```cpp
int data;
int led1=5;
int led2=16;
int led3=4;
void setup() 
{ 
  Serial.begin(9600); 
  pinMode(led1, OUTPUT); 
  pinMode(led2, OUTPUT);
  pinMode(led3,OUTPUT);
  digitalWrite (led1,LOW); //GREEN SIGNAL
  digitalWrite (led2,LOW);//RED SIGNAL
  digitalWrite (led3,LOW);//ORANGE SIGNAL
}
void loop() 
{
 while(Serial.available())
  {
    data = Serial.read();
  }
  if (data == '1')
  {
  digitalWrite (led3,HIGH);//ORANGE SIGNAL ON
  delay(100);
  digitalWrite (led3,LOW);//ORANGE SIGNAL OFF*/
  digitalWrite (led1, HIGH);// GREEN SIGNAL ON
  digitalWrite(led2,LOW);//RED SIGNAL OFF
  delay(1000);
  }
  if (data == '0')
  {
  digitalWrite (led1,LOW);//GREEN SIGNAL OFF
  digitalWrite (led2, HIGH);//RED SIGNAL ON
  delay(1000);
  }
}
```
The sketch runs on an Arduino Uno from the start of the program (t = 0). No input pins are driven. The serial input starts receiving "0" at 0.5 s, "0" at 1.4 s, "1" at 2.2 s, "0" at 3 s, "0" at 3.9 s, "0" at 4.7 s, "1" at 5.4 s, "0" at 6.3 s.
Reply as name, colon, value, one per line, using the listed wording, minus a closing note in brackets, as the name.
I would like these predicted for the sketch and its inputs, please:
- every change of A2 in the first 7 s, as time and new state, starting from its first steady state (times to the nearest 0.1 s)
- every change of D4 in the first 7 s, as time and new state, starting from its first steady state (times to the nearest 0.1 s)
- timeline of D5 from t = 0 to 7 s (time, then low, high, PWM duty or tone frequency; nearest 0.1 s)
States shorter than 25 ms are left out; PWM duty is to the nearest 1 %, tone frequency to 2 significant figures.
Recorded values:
every change of A2 in the first 7 s, as time and new state, starting from its first steady state: 0 s low; 0.5 s high; 2.6 s low; 3.6 s high; 5.7 s low; 6.7 s high
every change of D4 in the first 7 s, as time and new state, starting from its first steady state: 0 s low; 2.5 s high; 2.6 s low; 5.6 s high; 5.7 s low
timeline of D5 from t = 0 to 7 s: 0 s low; 2.6 s high; 3.6 s low; 5.7 s high; 6.7 s low
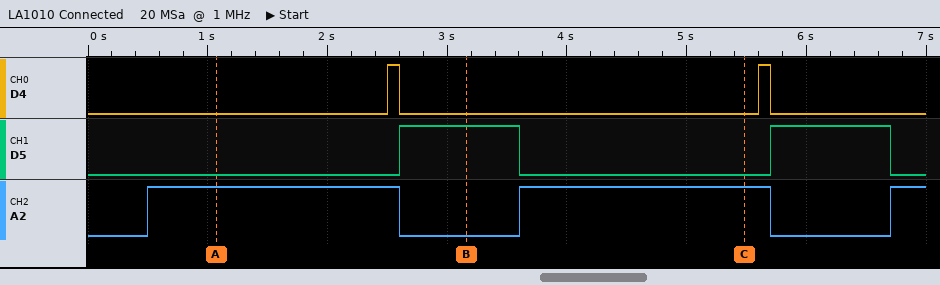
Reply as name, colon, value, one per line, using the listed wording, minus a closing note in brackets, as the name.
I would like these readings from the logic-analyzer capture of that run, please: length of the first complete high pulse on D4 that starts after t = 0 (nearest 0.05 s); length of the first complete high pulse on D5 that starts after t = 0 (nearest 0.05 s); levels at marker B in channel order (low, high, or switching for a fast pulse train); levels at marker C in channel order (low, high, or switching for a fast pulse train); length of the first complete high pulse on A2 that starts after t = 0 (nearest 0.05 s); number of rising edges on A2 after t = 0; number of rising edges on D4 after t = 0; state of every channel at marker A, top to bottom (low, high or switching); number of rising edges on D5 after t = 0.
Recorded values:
length of the first complete high pulse on D4 that starts after t = 0: 0.10 s
length of the first complete high pulse on D5 that starts after t = 0: 1.00 s
levels at marker B in channel order: D4 low, D5 high, A2 low
levels at marker C in channel order: D4 low, D5 low, A2 high
length of the first complete high pulse on A2 that starts after t = 0: 2.10 s
number of rising edges on A2 after t = 0: 3
number of rising edges on D4 after t = 0: 2
state of every channel at marker A, top to bottom: D4 low, D5 low, A2 high
number of rising edges on D5 after t = 0: 2
